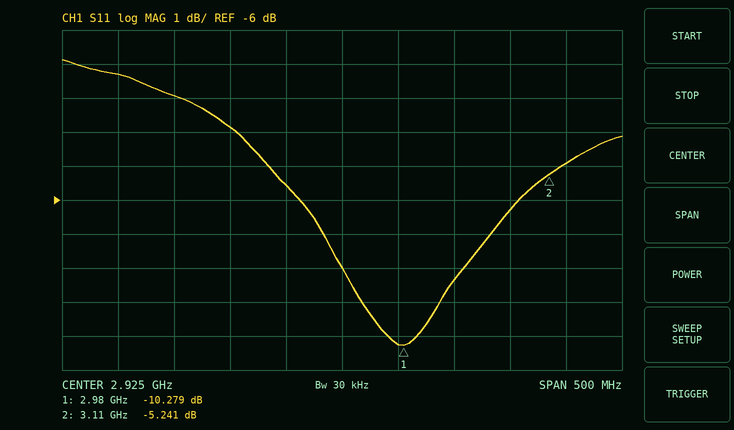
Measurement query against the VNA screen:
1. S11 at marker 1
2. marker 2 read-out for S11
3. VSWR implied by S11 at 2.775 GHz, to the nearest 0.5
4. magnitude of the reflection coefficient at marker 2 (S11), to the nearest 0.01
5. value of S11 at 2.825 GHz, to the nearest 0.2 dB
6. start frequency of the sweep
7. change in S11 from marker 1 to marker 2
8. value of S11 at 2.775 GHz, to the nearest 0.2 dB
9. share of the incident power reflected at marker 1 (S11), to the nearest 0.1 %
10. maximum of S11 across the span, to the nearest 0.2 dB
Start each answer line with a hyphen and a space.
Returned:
- -10.279 dB
- -5.241 dB
- 6.0
- 0.55
- -3.8 dB
- 2.675 GHz
- 5.038 dB
- -3.0 dB
- 9.4 %
- -1.8 dB
